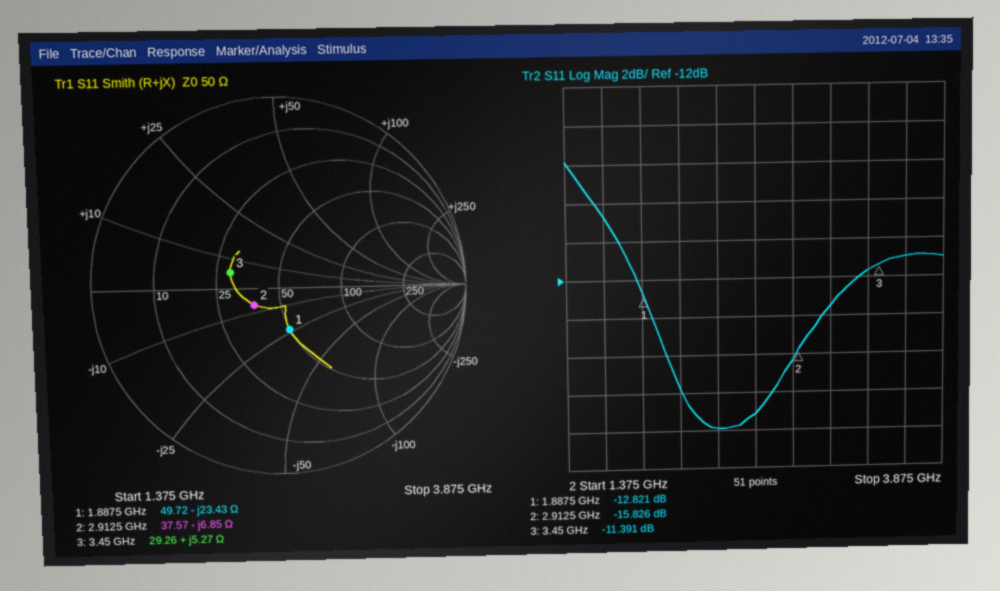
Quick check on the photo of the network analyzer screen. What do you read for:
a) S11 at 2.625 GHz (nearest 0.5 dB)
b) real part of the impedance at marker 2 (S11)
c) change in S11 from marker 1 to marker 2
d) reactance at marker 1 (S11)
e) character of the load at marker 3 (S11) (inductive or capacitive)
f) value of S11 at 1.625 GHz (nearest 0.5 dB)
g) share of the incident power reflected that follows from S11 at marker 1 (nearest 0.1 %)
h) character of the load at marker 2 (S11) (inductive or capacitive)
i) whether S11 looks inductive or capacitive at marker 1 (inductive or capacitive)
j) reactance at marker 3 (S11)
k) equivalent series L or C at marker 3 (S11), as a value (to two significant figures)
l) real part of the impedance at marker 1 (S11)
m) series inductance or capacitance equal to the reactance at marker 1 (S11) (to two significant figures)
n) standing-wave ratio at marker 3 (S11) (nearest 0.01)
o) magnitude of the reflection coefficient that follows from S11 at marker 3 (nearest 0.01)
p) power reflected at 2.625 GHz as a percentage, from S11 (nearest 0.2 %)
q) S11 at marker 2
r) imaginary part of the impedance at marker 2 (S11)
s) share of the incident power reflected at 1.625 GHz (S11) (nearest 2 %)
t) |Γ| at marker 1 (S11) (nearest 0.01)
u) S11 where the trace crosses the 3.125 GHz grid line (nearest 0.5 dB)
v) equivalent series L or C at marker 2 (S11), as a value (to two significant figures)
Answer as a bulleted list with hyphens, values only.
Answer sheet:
- -19.0 dB
- 37.57 Ω
- -3.005 dB
- -23.43 Ω
- inductive
- -8.5 dB
- 5.2 %
- capacitive
- capacitive
- +5.27 Ω
- 240 pH
- 49.72 Ω
- 3.6 pF
- 1.74
- 0.27
- 1.2 %
- -15.826 dB
- -6.85 Ω
- 14 %
- 0.23
- -13.5 dB
- 8.0 pF
